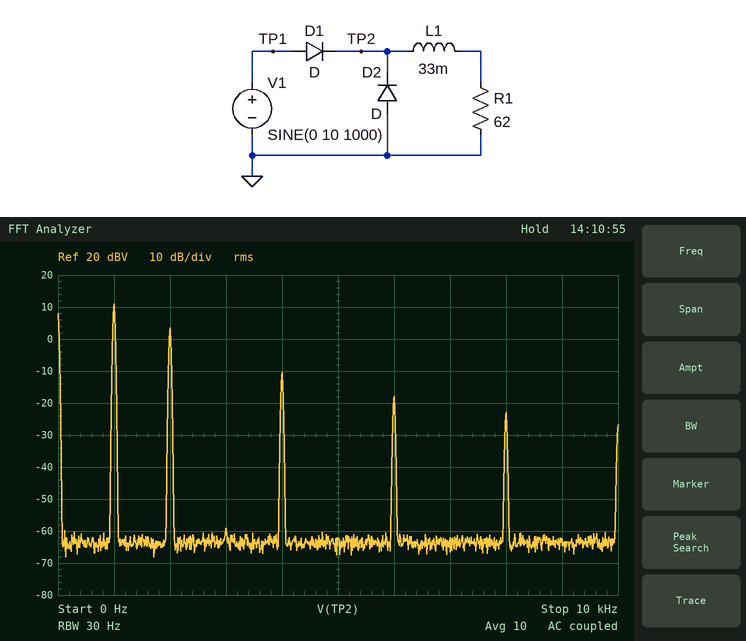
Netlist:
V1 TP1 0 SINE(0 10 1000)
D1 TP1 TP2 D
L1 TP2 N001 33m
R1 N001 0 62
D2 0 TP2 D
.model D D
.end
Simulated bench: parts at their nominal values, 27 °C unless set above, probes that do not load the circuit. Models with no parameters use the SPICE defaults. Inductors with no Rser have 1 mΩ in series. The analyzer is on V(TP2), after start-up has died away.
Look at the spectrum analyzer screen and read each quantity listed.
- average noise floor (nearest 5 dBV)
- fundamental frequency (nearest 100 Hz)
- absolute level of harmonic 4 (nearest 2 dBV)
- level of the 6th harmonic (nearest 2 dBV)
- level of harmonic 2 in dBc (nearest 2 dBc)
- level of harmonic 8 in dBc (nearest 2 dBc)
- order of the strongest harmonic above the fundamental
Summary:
-65 dBV
1.0 kHz
-10 dBV
-18 dBV
-8 dBc
-34 dBc
2
